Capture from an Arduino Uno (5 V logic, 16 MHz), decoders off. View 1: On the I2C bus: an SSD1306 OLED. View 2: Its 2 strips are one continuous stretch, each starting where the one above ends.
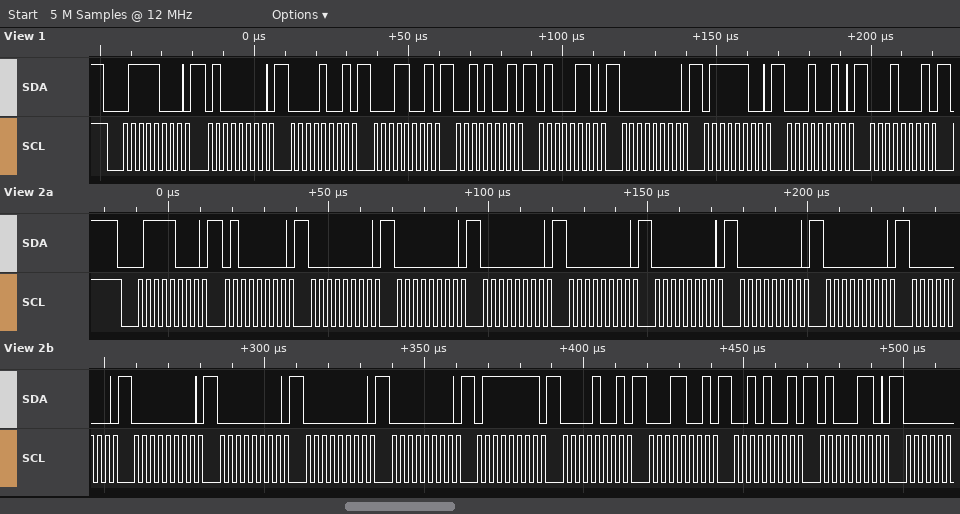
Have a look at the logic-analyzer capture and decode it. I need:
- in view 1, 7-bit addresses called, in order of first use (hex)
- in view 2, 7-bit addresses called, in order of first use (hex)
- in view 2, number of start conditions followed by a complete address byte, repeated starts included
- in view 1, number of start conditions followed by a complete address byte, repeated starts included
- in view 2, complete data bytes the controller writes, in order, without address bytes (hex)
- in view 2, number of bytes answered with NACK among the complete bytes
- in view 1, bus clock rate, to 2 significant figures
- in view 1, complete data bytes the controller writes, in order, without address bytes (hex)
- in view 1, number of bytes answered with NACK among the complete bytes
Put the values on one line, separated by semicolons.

0x3C; 0x3C; 1; 1; 40 00 00 00 00 00 00 00 00 00 00 00 00 7F 09 19 29 46; 0; 400 kHz; 40 09 19 29 46 00 7C 12 11; 0
